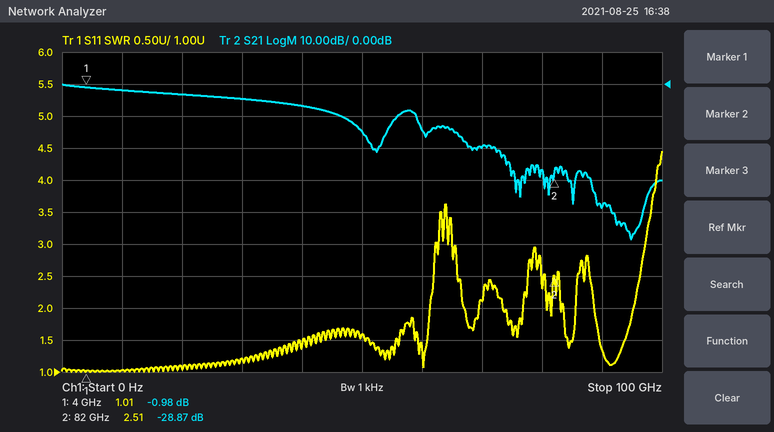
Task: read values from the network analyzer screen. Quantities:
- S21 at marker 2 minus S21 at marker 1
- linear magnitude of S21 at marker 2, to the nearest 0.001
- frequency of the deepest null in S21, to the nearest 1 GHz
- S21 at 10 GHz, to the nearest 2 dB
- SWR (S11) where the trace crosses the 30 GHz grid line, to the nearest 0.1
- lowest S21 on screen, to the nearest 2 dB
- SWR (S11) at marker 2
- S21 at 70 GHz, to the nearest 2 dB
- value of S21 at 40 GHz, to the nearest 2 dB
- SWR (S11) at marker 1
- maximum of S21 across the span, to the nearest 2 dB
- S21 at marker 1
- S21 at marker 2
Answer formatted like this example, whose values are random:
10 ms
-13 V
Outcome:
-27.89 dB
0.036
95 GHz
-2 dB
1.2
-48 dB
2.51
-20 dB
-6 dB
1.01
0 dB
-0.98 dB
-28.87 dB
